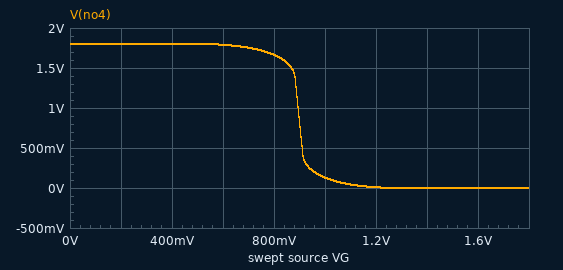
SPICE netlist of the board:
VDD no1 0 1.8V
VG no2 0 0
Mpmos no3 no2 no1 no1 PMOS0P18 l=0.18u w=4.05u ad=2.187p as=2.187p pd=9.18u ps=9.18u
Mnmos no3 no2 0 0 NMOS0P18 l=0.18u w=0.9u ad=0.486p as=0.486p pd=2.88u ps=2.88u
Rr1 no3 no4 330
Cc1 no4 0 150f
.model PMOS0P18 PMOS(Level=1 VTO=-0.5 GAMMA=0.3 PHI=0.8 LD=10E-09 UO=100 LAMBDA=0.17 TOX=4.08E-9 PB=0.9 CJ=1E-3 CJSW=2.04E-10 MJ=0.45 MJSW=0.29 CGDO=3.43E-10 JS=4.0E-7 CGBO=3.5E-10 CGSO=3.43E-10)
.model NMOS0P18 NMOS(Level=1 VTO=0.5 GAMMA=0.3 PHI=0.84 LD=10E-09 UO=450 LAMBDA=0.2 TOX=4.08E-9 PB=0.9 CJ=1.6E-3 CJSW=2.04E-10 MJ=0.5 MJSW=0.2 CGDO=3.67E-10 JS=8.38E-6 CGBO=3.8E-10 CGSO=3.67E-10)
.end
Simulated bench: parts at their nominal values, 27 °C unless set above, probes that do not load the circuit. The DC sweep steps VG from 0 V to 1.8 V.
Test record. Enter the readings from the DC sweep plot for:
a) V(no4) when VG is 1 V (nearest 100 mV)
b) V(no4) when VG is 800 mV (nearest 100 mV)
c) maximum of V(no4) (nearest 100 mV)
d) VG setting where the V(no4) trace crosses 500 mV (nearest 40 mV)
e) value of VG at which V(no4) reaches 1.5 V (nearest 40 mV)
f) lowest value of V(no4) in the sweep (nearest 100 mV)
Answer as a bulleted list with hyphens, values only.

- 100 mV
- 1.7 V
- 1.8 V
- 920 mV
- 880 mV
- 0 V
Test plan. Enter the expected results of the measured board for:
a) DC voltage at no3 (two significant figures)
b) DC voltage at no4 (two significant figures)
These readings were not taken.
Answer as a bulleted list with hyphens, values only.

- 1.8 V
- 1.8 V
